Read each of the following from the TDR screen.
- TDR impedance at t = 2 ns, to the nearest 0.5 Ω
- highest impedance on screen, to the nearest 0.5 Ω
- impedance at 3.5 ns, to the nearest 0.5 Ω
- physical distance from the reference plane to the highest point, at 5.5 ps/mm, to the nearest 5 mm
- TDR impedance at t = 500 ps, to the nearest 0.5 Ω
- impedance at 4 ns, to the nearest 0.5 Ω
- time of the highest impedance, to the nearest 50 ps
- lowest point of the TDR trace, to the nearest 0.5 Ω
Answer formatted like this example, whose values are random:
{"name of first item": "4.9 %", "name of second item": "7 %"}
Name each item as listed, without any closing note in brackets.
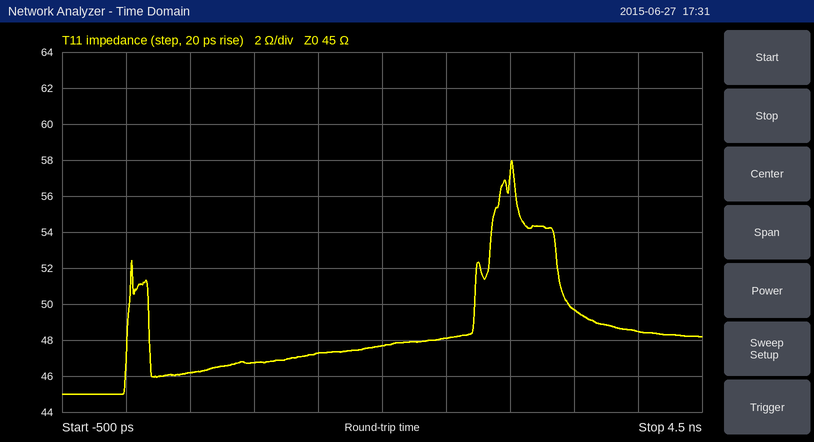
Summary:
{"TDR impedance at t = 2 ns, to the nearest 0.5 Ω": "47.5 Ω", "highest impedance on screen, to the nearest 0.5 Ω": "58.0 Ω", "impedance at 3.5 ns, to the nearest 0.5 Ω": "49.5 Ω", "physical distance from the reference plane to the highest point, at 5.5 ps/mm, to the nearest 5 mm": "275 mm", "TDR impedance at t = 500 ps, to the nearest 0.5 Ω": "46.0 Ω", "impedance at 4 ns, to the nearest 0.5 Ω": "48.5 Ω", "time of the highest impedance, to the nearest 50 ps": "3.00 ns", "lowest point of the TDR trace, to the nearest 0.5 Ω": "45.0 Ω"}
